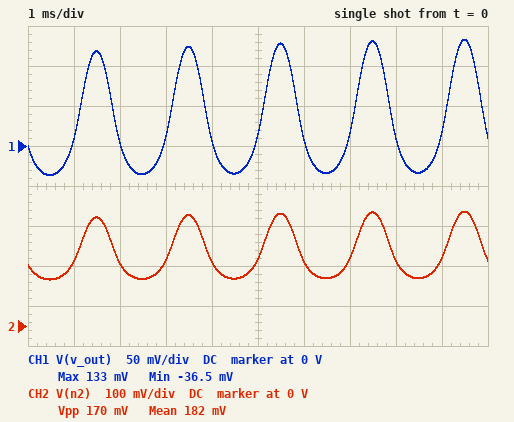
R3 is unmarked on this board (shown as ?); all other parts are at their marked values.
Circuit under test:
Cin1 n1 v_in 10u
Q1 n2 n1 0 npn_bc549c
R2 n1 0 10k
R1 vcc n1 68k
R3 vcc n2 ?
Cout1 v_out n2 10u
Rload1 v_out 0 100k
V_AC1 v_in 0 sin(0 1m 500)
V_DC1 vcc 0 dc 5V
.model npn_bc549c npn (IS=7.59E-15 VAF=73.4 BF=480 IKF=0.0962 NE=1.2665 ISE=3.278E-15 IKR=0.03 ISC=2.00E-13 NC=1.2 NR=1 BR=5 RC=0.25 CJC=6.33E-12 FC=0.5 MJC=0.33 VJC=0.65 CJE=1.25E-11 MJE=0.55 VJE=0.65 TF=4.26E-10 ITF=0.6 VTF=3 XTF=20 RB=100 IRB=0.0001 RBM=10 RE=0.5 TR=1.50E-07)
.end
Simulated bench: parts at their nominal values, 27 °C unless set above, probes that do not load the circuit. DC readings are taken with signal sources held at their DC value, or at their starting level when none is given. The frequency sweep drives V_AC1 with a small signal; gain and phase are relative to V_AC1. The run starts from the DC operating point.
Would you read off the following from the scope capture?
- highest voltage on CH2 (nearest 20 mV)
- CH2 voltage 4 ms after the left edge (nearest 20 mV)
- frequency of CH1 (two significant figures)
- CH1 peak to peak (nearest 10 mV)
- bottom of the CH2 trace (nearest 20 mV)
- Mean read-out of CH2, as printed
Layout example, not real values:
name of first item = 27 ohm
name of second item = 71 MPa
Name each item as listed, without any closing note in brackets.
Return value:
highest voltage on CH2 = 280 mV
CH2 voltage 4 ms after the left edge = 160 mV
frequency of CH1 = 500 Hz
CH1 peak to peak = 170 mV
bottom of the CH2 trace = 120 mV
Mean read-out of CH2, as printed = 182 mV
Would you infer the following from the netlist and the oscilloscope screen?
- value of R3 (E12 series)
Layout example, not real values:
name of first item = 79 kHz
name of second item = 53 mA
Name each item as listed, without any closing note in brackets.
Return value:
value of R3 = 22 kΩ
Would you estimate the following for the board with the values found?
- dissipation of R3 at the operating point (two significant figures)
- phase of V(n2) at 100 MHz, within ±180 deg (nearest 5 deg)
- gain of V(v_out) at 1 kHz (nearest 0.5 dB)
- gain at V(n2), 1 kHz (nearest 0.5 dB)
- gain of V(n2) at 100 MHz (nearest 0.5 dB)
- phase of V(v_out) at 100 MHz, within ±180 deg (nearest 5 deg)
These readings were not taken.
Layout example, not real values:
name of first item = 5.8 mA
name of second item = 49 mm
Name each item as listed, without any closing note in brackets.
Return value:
dissipation of R3 at the operating point = 1.1 mW
phase of V(n2) at 100 MHz, within ±180 deg = 0 deg
gain of V(v_out) at 1 kHz = 36.0 dB
gain at V(n2), 1 kHz = 36.0 dB
gain of V(n2) at 100 MHz = -5.0 dB
phase of V(v_out) at 100 MHz, within ±180 deg = 0 deg
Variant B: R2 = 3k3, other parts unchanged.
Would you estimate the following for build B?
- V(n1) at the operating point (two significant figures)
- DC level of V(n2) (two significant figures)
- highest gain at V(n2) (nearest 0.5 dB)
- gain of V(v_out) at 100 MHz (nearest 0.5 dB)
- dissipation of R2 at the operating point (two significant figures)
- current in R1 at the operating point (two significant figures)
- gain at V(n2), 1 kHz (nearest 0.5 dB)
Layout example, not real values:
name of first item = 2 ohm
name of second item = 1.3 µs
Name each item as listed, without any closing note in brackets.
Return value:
V(n1) at the operating point = 230 mV
DC level of V(n2) = 5.0 V
highest gain at V(n2) = -0.5 dB
gain of V(v_out) at 100 MHz = -3.0 dB
dissipation of R2 at the operating point = 16 µW
current in R1 at the operating point = 70 µA
gain at V(n2), 1 kHz = -69.0 dB
